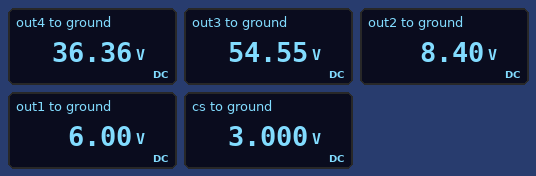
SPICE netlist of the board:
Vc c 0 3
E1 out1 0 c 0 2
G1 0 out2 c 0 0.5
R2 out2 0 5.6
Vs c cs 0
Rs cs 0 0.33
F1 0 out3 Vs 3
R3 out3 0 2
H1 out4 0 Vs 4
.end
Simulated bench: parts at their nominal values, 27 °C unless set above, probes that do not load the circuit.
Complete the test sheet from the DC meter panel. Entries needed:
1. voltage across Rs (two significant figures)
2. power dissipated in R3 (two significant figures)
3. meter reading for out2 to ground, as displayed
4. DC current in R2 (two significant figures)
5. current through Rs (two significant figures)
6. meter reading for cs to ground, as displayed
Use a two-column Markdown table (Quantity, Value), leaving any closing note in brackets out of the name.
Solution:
| Quantity | Value |
|---|---|
| voltage across Rs | 3.0 V |
| power dissipated in R3 | 1.5 kW |
| meter reading for out2 to ground, as displayed | 8.40 V |
| DC current in R2 | 1.5 A |
| current through Rs | 9.1 A |
| meter reading for cs to ground, as displayed | 3.000 V |
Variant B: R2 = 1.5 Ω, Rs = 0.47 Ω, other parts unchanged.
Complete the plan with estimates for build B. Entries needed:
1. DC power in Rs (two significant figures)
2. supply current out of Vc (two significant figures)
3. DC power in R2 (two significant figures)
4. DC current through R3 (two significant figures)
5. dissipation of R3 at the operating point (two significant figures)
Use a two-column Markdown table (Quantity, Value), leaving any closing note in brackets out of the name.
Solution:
| Quantity | Value |
|---|---|
| DC power in Rs | 19 W |
| supply current out of Vc | 6.4 A |
| DC power in R2 | 3.4 W |
| DC current through R3 | 19 A |
| dissipation of R3 at the operating point | 730 W |
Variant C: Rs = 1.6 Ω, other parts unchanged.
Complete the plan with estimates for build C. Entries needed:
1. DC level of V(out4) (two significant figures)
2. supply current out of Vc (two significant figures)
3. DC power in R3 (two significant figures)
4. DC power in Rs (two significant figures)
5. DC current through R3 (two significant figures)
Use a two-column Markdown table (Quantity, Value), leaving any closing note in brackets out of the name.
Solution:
| Quantity | Value |
|---|---|
| DC level of V(out4) | 7.5 V |
| supply current out of Vc | 1.9 A |
| DC power in R3 | 63 W |
| DC power in Rs | 5.6 W |
| DC current through R3 | 5.6 A |
